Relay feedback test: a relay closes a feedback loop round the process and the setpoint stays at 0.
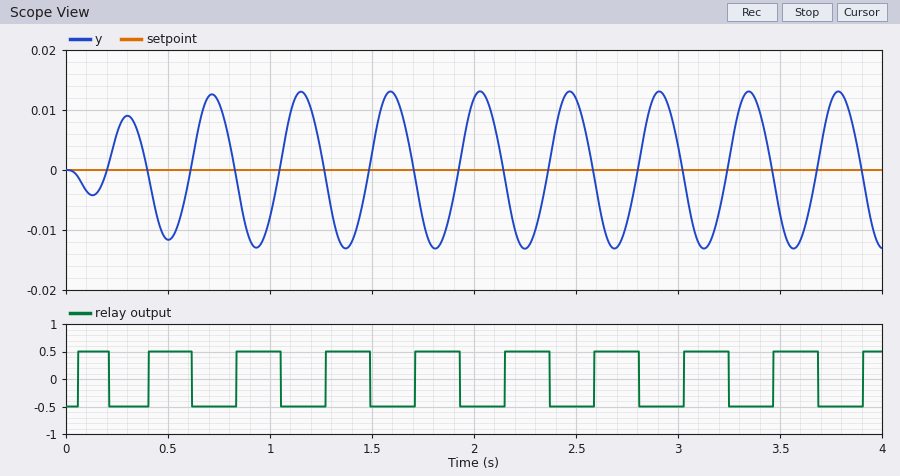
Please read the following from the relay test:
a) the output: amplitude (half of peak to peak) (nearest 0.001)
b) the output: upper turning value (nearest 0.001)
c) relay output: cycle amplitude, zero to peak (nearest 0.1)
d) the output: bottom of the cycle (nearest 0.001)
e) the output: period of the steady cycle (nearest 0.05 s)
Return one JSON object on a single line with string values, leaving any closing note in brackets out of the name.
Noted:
{"the output: amplitude (half of peak to peak)": "0.013", "the output: upper turning value": "0.013", "relay output: cycle amplitude, zero to peak": "0.5", "the output: bottom of the cycle": "-0.013", "the output: period of the steady cycle": "0.45 s"}
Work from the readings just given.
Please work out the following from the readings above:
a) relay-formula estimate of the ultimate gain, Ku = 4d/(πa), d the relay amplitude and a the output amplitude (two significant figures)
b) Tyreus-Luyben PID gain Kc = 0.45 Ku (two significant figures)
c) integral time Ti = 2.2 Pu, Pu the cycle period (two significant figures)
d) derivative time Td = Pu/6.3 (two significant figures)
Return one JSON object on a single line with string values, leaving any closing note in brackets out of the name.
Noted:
{"relay-formula estimate of the ultimate gain, Ku = 4d/(πa), d the relay amplitude and a the output amplitude": "49", "Tyreus-Luyben PID gain Kc = 0.45 Ku": "22", "integral time Ti = 2.2 Pu, Pu the cycle period": "0.99 s", "derivative time Td = Pu/6.3": "0.071 s"}
